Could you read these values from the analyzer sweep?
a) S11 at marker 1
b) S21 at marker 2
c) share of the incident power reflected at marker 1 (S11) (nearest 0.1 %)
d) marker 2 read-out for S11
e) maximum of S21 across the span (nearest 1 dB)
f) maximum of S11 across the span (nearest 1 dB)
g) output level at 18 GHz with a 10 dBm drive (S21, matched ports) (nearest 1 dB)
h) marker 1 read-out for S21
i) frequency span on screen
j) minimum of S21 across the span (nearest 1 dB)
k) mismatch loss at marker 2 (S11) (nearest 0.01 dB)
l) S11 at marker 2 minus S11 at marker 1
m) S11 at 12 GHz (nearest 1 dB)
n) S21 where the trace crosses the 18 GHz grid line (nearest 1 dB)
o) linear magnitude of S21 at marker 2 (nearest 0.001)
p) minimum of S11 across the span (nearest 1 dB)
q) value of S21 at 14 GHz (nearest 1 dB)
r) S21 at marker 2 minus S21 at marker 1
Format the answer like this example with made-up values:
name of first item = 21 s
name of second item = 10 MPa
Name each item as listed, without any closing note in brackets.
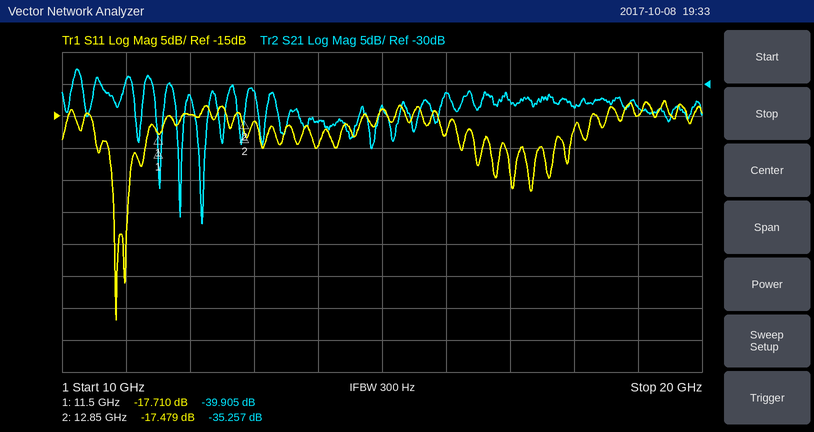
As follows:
S11 at marker 1 = -17.710 dB
S21 at marker 2 = -35.257 dB
share of the incident power reflected at marker 1 (S11) = 1.7 %
marker 2 read-out for S11 = -17.479 dB
maximum of S21 across the span = -28 dB
maximum of S11 across the span = -13 dB
output level at 18 GHz with a 10 dBm drive (S21, matched ports) = -24 dBm
marker 1 read-out for S21 = -39.905 dB
frequency span on screen = 10 GHz
minimum of S21 across the span = -52 dB
mismatch loss at marker 2 (S11) = 0.08 dB
S11 at marker 2 minus S11 at marker 1 = 0.231 dB
S11 at 12 GHz = -15 dB
S21 where the trace crosses the 18 GHz grid line = -34 dB
linear magnitude of S21 at marker 2 = 0.017
minimum of S11 across the span = -47 dB
value of S21 at 14 GHz = -36 dB
S21 at marker 2 minus S21 at marker 1 = 4.648 dB
